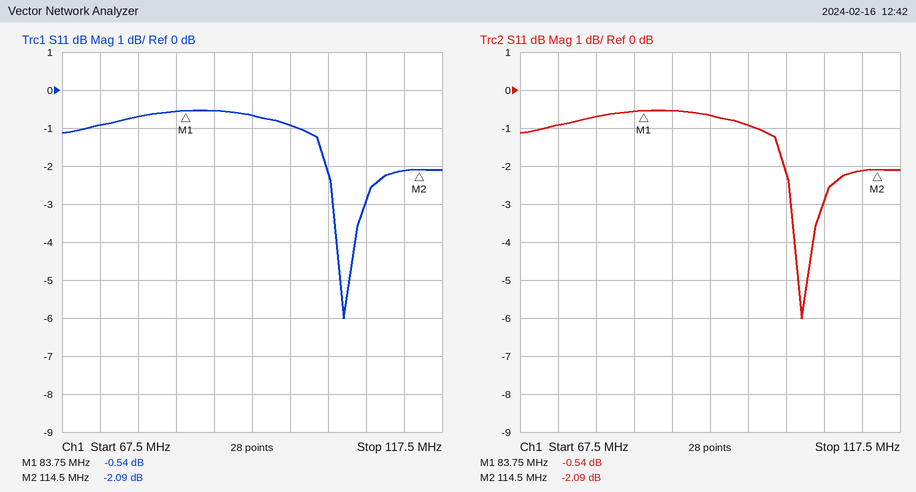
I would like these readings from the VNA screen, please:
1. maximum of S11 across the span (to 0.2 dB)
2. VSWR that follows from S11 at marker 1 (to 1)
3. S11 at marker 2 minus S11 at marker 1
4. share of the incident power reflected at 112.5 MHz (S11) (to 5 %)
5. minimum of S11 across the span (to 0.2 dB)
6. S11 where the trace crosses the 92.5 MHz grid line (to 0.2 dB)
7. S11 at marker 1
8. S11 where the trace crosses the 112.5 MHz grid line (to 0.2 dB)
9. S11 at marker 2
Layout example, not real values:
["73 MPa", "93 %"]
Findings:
["-0.6 dB", "32", "-1.55 dB", "60 %", "-6.0 dB", "-0.6 dB", "-0.54 dB", "-2.2 dB", "-2.09 dB"]
